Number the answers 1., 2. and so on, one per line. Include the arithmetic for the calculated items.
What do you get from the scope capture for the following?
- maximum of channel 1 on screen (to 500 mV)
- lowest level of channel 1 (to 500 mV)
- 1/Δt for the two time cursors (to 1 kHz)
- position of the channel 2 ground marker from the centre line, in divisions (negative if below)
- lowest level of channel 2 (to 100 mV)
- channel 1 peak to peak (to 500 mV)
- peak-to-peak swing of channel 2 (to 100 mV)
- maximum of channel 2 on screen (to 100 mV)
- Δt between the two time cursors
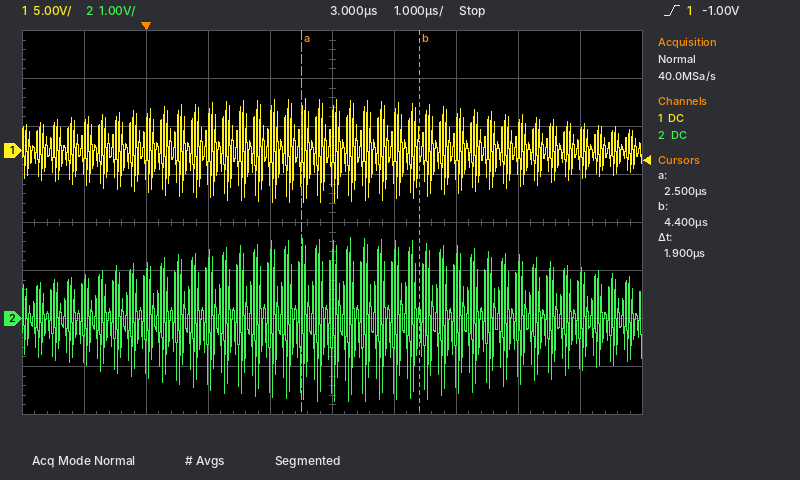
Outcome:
1. 5.5 V
2. -5.5 V
3. 1 / 1.9 µs ≈ 526 kHz
4. -2.0 div
5. -1.7 V
6. 5.5 V − (-5.5 V) = 11.0 V
7. 1.7 V − (-1.7 V) = 3.4 V
8. 1.7 V
9. 1.9 µs
